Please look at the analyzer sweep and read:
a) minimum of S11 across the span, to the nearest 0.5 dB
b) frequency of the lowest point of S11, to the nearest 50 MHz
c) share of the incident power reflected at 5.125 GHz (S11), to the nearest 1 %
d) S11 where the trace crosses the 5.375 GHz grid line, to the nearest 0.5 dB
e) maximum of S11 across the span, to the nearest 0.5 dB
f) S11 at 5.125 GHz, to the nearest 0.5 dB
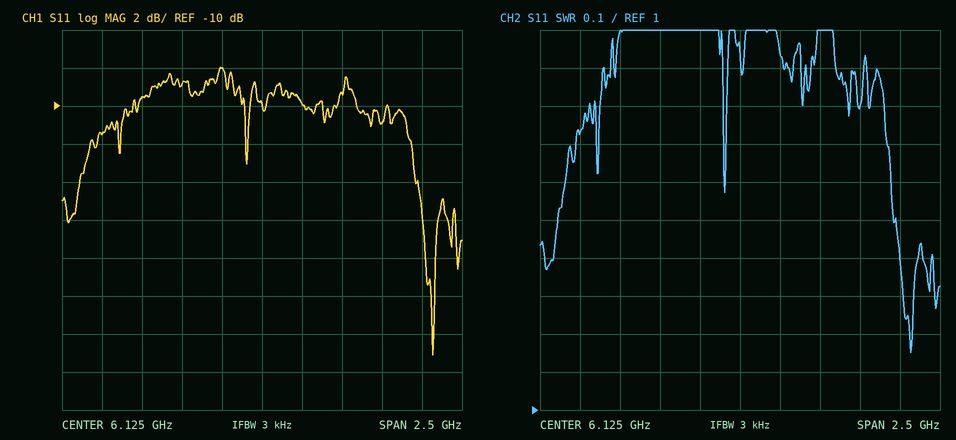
-23.0 dB
7.20 GHz
7 %
-9.5 dB
-8.0 dB
-11.5 dB
